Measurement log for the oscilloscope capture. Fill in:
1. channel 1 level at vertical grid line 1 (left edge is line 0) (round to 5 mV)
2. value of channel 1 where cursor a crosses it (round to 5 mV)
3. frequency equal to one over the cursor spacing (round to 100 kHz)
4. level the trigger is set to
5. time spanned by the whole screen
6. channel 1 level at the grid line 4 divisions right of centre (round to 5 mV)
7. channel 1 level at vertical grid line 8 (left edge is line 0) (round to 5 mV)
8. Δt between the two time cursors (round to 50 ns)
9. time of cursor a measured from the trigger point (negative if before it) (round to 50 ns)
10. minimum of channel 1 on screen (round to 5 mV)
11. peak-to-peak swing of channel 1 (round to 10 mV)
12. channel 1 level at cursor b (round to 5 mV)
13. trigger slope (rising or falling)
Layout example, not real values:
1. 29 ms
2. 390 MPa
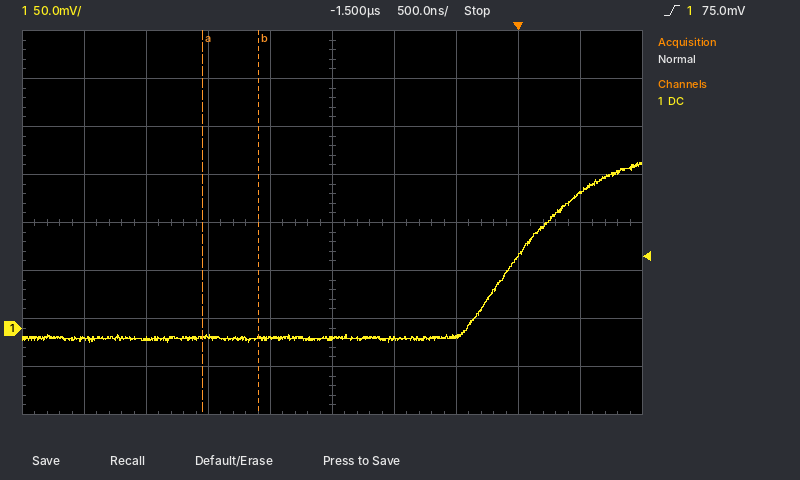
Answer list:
1. -10 mV
2. -10 mV
3. 2.2 MHz
4. 75.0 mV
5. 5 µs
6. 140 mV
7. 75 mV
8. 450 ns
9. -2.55 µs
10. -15 mV
11. 190 mV
12. -10 mV
13. rising
